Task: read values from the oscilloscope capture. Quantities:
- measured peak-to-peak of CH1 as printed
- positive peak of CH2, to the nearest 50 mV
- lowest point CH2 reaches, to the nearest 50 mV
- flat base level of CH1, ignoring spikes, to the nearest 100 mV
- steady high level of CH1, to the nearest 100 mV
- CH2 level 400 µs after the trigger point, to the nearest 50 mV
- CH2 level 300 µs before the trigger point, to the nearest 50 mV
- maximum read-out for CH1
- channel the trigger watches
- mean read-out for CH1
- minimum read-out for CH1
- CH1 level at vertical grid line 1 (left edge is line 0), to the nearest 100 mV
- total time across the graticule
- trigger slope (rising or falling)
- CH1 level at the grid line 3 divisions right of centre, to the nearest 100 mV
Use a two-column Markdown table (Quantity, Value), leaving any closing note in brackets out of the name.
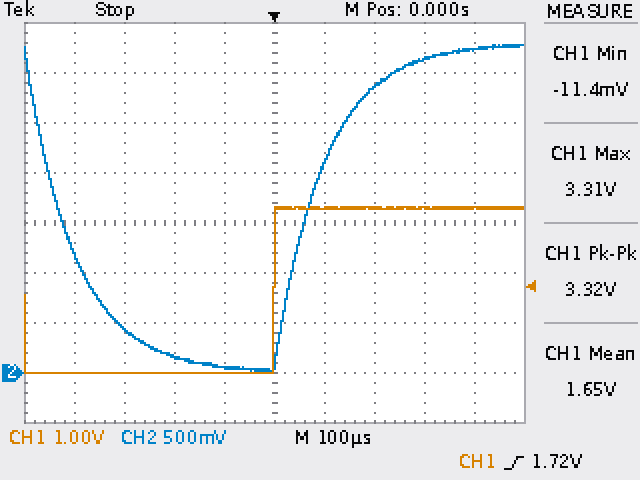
| Quantity | Value |
|---|---|
| measured peak-to-peak of CH1 as printed | 3.32 V |
| positive peak of CH2, to the nearest 50 mV | 3.30 V |
| lowest point CH2 reaches, to the nearest 50 mV | 0 mV |
| flat base level of CH1, ignoring spikes, to the nearest 100 mV | 0.0 V |
| steady high level of CH1, to the nearest 100 mV | 3.3 V |
| CH2 level 400 µs after the trigger point, to the nearest 50 mV | 3.25 V |
| CH2 level 300 µs before the trigger point, to the nearest 50 mV | 450 mV |
| maximum read-out for CH1 | 3.31 V |
| channel the trigger watches | CH1 |
| mean read-out for CH1 | 1.65 V |
| minimum read-out for CH1 | -11.4 mV |
| CH1 level at vertical grid line 1 (left edge is line 0), to the nearest 100 mV | 0.0 V |
| total time across the graticule | 1 ms |
| trigger slope | rising |
| CH1 level at the grid line 3 divisions right of centre, to the nearest 100 mV | 3.3 V |
